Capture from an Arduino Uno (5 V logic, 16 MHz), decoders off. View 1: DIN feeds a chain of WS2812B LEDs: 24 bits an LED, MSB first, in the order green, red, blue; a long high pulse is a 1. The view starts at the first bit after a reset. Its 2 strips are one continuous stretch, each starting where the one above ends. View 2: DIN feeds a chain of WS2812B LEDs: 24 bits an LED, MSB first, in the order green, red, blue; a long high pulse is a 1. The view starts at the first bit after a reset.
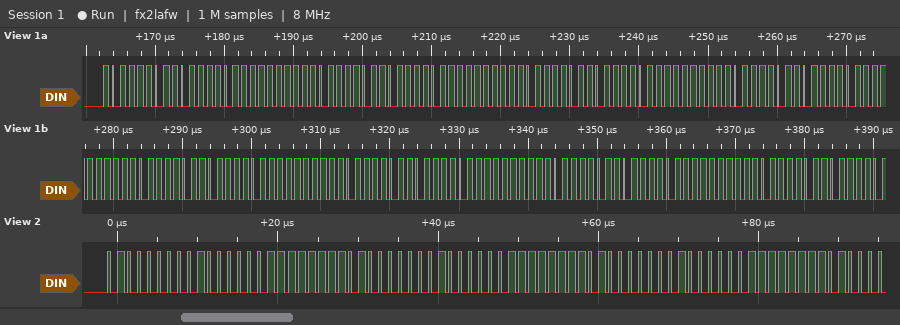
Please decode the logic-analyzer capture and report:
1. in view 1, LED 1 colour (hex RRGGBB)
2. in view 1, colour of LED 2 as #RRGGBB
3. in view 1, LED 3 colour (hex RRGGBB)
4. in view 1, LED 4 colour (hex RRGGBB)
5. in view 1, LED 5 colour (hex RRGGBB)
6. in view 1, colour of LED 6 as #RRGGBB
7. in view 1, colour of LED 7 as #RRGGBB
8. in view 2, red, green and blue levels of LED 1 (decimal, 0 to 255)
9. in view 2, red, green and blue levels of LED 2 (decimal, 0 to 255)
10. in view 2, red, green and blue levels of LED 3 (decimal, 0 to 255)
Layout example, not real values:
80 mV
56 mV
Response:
#BDBDFF
#BDBDFF
#BDBDFF
#BDBDFF
#BDBDFF
#BDBDFF
#BDBDFF
64, 64, 255
64, 64, 255
64, 64, 255
